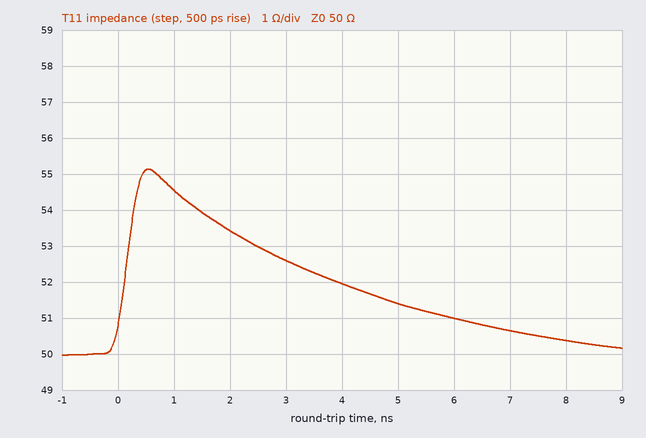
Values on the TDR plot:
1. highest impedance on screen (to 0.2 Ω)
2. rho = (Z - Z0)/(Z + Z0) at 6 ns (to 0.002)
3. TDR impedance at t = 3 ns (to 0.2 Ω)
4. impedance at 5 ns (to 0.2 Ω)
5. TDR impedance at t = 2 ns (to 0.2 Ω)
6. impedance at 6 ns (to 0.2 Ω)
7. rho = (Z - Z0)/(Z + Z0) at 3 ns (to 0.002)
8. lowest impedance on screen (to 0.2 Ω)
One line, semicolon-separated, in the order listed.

55.2 Ω; +0.010; 52.6 Ω; 51.4 Ω; 53.4 Ω; 51.0 Ω; +0.026; 50.0 Ω
